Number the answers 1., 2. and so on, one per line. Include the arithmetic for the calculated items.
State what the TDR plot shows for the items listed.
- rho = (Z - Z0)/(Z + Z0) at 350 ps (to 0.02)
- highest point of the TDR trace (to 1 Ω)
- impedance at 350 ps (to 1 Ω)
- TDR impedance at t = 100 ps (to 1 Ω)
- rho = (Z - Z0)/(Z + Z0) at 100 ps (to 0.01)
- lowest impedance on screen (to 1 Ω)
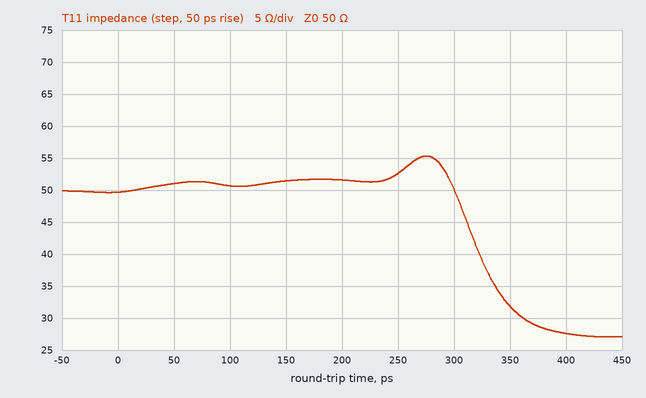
1. (32 − 50)/(32 + 50) ≈ -0.22
2. 55 Ω
3. 32 Ω
4. 51 Ω
5. (51 − 50)/(51 + 50) ≈ +0.01
6. 27 Ω
